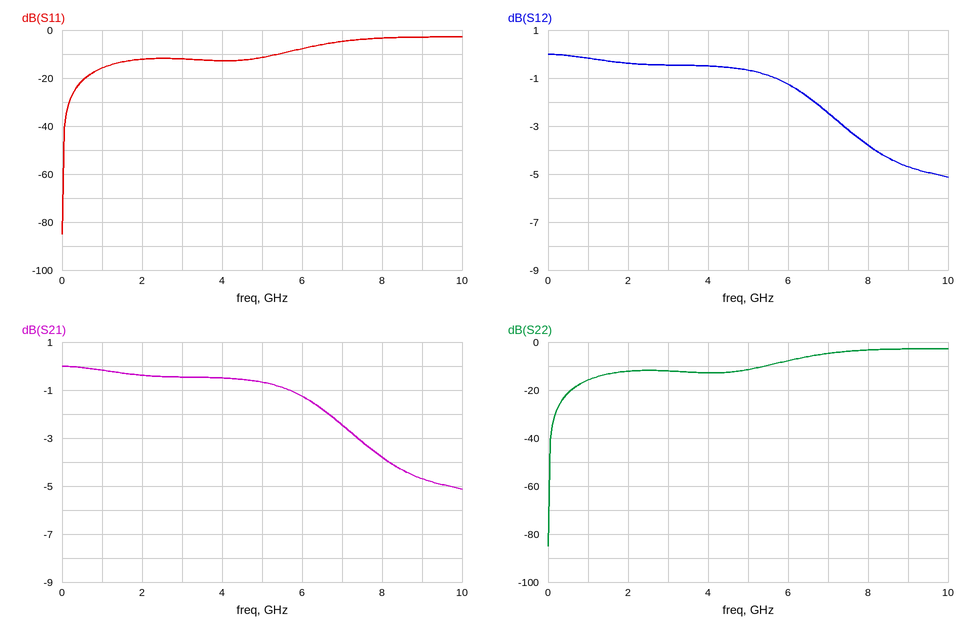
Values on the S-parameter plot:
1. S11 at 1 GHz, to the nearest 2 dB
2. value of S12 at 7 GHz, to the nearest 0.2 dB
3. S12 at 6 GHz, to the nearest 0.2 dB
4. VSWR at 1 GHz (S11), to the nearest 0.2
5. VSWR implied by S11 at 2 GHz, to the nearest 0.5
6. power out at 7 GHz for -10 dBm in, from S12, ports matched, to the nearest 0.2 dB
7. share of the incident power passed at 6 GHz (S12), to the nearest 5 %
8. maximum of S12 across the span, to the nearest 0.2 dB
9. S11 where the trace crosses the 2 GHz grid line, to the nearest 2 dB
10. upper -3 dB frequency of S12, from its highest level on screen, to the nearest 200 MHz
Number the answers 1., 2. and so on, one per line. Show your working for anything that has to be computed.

1. -16 dB
2. -2.4 dB
3. -1.2 dB
4. |Γ| = 10^(-16/20) = 0.1585; VSWR = (1 + 0.1585)/(1 − 0.1585) ≈ 1.4
5. |Γ| = 10^(-12/20) = 0.2512; VSWR = (1 + 0.2512)/(1 − 0.2512) ≈ 1.67, so 1.5 to the nearest 0.5
6. -10 dBm + (-2.4 dB) = -12.4 dBm
7. 10^(-1.2/10) ≈ 75.9 %, so 75 % to the nearest 5 %
8. 0.0 dB
9. -12 dB
10. 7.4 GHz
